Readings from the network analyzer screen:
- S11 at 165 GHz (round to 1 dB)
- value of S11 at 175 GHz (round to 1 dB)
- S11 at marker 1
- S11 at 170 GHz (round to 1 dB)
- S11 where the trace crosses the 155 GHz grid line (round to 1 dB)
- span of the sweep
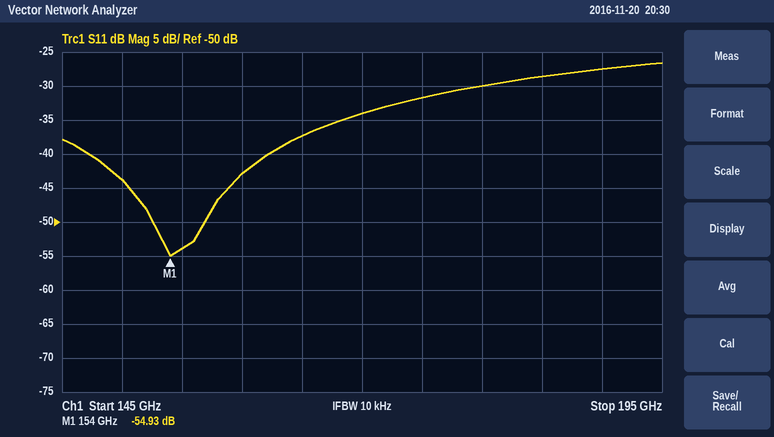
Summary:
-37 dB
-32 dB
-54.93 dB
-34 dB
-54 dB
50 GHz
